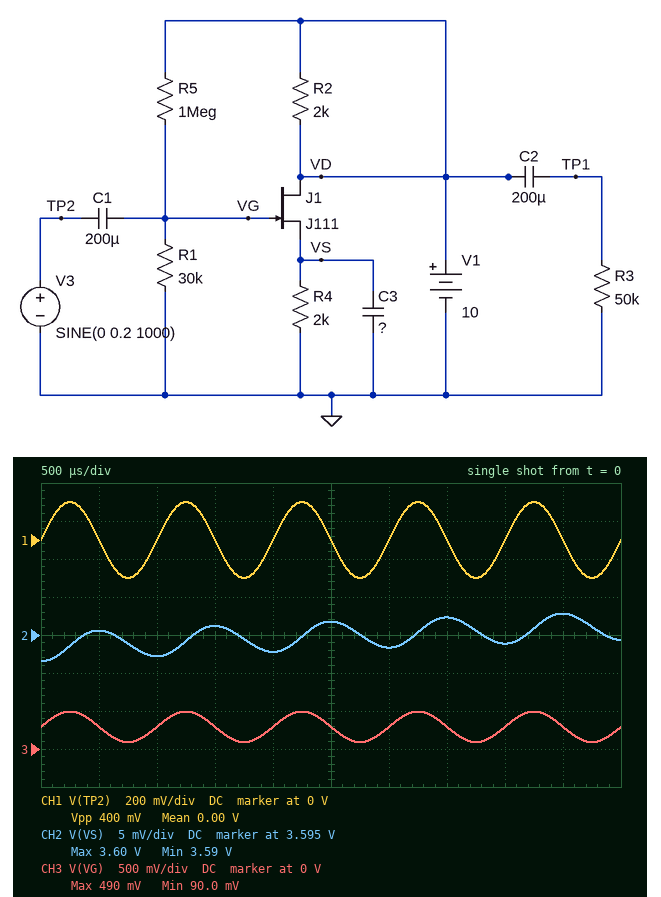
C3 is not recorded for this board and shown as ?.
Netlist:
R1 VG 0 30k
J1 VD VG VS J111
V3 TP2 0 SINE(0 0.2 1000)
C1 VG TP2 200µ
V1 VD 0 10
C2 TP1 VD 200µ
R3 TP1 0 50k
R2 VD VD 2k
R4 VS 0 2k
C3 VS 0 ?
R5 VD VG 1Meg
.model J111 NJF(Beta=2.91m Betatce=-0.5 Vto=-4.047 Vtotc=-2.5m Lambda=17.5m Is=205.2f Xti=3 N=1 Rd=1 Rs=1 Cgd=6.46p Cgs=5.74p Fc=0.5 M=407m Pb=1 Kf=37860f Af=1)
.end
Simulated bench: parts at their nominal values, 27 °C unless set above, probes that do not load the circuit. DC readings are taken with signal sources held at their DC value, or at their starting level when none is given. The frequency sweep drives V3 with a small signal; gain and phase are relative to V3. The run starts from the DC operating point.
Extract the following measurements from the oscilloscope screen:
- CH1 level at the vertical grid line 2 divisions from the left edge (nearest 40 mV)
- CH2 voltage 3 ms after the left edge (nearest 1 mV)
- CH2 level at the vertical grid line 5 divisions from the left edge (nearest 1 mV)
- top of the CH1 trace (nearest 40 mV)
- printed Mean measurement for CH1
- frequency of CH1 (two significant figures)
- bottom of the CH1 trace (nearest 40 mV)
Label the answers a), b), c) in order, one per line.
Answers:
a) 0 V
b) 3.593 V
c) 3.597 V
d) 200 mV
e) 0.00 V
f) 1.0 kHz
g) -200 mV
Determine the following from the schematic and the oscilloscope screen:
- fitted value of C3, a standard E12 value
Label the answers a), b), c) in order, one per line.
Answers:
a) 82 µF
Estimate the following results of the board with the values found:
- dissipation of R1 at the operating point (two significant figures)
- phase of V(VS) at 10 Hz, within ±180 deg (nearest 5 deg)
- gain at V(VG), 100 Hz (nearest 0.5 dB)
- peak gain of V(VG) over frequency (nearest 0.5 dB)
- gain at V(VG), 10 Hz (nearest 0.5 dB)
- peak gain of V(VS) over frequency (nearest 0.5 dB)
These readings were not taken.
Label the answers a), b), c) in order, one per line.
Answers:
a) 2.8 µW
b) -45 deg
c) 0 dB
d) 0 dB
e) 0 dB
f) -1.0 dB
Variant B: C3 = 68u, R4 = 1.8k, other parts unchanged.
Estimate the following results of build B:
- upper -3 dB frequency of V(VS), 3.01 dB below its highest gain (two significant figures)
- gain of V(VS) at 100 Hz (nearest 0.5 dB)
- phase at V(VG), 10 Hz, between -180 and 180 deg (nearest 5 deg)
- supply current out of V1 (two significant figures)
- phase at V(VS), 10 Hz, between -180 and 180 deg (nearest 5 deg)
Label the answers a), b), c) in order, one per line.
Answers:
a) 13 Hz
b) -18.5 dB
c) 0 deg
d) 2.0 mA
e) -35 deg
